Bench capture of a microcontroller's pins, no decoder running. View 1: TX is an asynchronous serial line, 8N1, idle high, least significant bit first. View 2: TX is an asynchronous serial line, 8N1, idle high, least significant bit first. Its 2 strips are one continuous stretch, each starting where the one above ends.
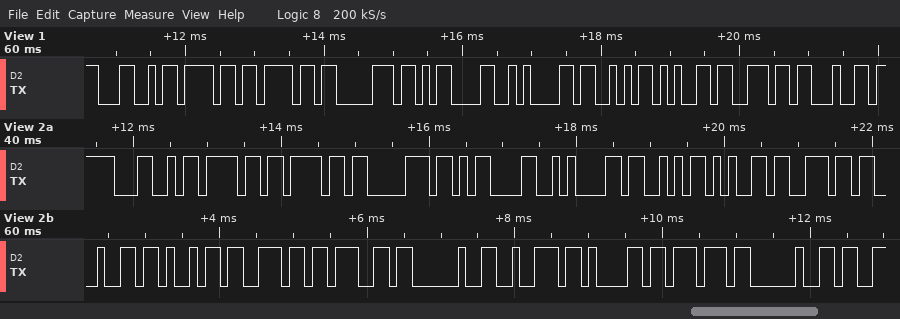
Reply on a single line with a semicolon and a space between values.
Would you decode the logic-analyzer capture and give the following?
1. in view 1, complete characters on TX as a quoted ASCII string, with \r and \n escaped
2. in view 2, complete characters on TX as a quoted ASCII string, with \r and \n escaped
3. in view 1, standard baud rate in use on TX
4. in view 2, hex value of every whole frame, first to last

"Loop\r\nSend"; "Loop\r\nSending raw "; 9600 baud; 0x4C 0x6F 0x6F 0x70 0x0D 0x0A 0x53 0x65 0x6E 0x64 0x69 0x6E 0x67 0x20 0x72 0x61 0x77 0x20
